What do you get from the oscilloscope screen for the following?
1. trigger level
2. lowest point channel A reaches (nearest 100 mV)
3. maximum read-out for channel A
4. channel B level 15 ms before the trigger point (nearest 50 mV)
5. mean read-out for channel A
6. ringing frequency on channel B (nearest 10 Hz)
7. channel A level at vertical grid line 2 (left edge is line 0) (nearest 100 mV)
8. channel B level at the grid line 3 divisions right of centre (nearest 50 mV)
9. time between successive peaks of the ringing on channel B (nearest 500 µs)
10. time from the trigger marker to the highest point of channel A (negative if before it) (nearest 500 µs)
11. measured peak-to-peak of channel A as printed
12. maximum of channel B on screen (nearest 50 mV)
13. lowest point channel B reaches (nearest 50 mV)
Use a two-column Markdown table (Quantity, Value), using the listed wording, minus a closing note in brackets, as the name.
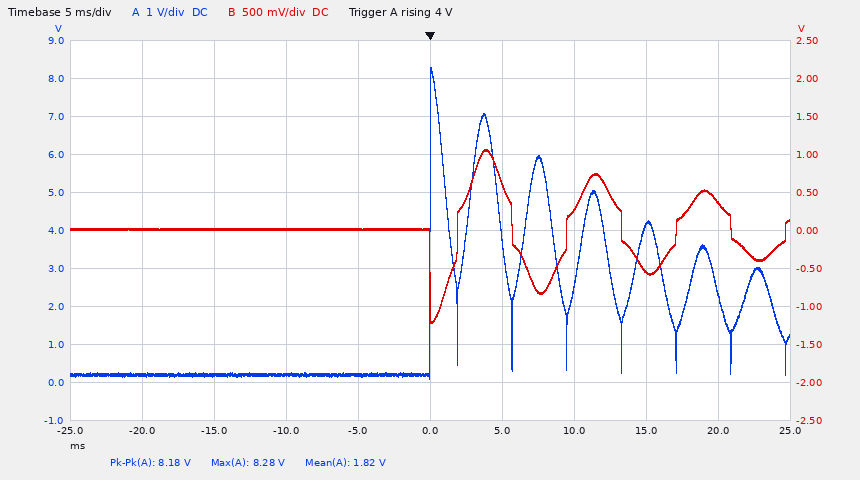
| Quantity | Value |
|---|---|
| trigger level | 4 V |
| lowest point channel A reaches | 100 mV |
| maximum read-out for channel A | 8.28 V |
| channel B level 15 ms before the trigger point | 0 mV |
| mean read-out for channel A | 1.82 V |
| ringing frequency on channel B | 130 Hz |
| channel A level at vertical grid line 2 (left edge is line 0) | 200 mV |
| channel B level at the grid line 3 divisions right of centre | -550 mV |
| time between successive peaks of the ringing on channel B | 7.5 ms |
| time from the trigger marker to the highest point of channel A (negative if before it) | 0.0 ms |
| measured peak-to-peak of channel A as printed | 8.18 V |
| maximum of channel B on screen | 1.05 V |
| lowest point channel B reaches | -1.20 V |
